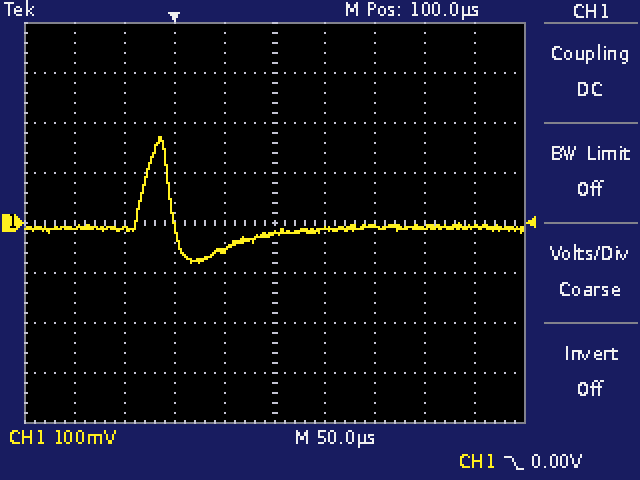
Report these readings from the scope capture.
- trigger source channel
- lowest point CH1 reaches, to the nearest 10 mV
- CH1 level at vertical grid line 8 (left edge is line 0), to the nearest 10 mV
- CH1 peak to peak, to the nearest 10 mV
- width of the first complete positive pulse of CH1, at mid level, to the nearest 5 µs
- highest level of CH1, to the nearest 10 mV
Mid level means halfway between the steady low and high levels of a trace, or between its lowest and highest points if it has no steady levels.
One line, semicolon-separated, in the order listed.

CH1; -80 mV; -10 mV; 250 mV; 30 µs; 170 mV
